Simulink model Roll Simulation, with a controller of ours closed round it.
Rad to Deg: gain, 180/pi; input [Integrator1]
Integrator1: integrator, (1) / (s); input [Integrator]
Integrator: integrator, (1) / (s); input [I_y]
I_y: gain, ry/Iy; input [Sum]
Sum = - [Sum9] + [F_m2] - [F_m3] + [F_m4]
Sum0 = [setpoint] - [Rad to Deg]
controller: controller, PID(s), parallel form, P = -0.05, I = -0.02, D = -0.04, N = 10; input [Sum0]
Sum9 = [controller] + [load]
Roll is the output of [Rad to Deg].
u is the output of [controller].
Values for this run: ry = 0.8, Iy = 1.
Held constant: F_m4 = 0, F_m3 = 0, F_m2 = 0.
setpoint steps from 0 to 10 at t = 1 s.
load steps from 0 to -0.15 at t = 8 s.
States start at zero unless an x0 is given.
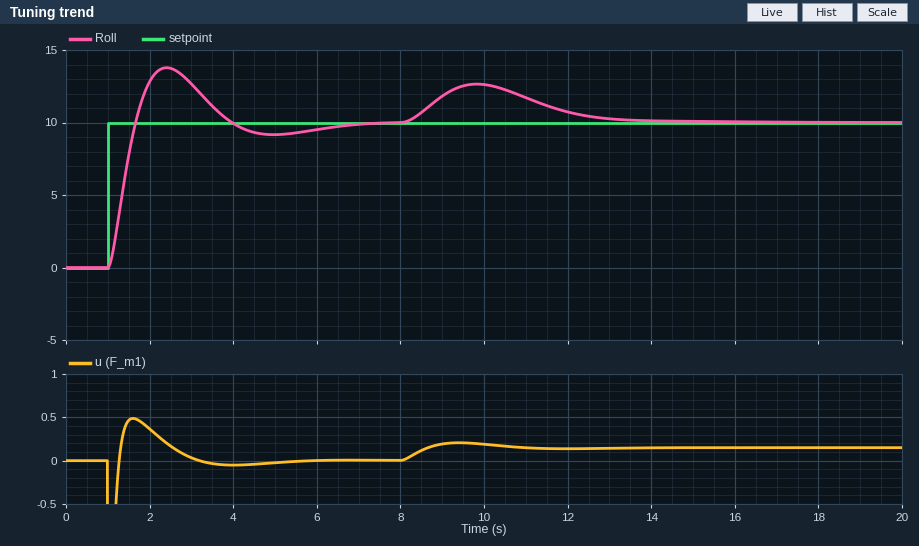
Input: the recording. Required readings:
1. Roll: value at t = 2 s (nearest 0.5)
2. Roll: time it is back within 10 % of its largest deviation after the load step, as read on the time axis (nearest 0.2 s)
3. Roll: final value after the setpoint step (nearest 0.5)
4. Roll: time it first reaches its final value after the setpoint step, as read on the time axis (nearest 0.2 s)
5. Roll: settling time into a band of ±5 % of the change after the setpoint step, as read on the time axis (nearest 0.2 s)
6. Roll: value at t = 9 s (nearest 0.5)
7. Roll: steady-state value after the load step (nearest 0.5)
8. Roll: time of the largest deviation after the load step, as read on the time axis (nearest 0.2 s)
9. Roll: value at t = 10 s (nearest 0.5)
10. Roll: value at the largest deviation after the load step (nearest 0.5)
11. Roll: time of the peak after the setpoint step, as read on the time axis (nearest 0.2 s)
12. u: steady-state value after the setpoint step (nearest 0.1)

13.0
13.0 s
10.0
1.6 s
6.0 s
12.0
10.0
9.8 s
12.5
12.5
2.4 s
0.0
